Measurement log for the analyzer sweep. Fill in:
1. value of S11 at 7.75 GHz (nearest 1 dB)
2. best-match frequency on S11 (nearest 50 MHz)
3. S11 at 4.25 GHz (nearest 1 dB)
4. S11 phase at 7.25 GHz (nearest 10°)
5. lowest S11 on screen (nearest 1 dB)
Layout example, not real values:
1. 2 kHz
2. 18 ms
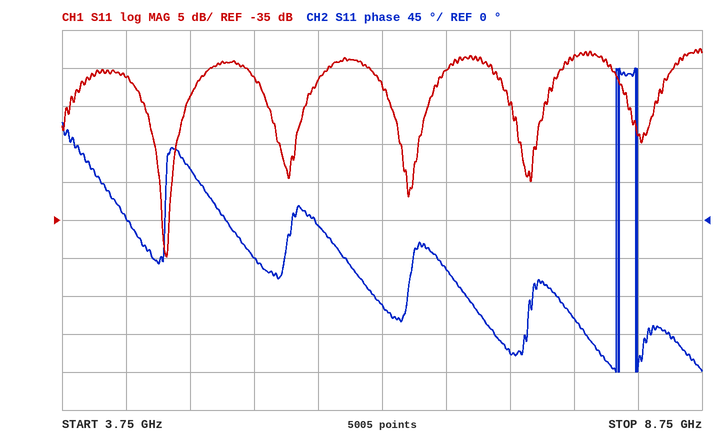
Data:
1. -13 dB
2. 4.55 GHz
3. -16 dB
4. -160°
5. -40 dB
